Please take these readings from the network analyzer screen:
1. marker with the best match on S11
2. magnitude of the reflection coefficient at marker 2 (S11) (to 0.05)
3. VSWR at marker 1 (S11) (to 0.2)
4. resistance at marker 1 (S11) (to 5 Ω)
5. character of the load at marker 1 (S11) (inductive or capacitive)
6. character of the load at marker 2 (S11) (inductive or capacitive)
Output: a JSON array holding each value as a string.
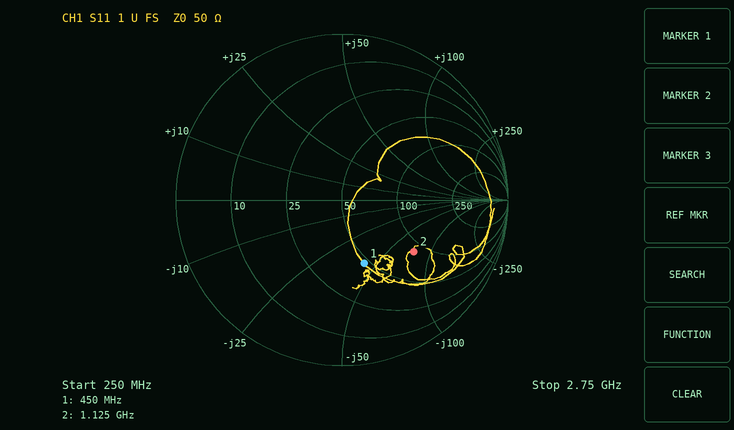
["marker 1", "0.55", "2.4", "45 Ω", "capacitive", "capacitive"]
